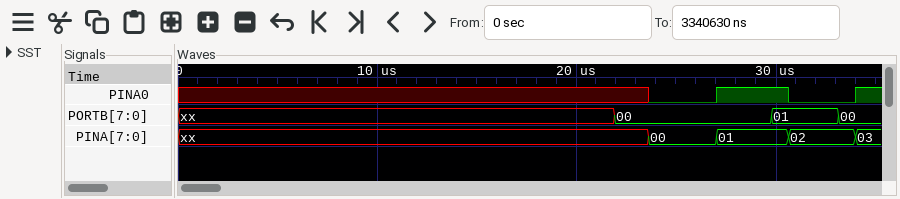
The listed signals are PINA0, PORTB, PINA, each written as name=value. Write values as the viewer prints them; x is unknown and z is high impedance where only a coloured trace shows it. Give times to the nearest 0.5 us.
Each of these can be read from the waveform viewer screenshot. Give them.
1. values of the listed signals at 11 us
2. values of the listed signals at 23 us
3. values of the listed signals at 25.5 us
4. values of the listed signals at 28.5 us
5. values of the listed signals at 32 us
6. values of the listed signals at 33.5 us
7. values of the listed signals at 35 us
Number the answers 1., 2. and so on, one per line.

1. PINA0=x, PORTB=xx, PINA=xx
2. PINA0=x, PORTB=00, PINA=xx
3. PINA0=0, PORTB=00, PINA=00
4. PINA0=1, PORTB=00, PINA=01
5. PINA0=0, PORTB=01, PINA=02
6. PINA0=0, PORTB=00, PINA=02
7. PINA0=1, PORTB=00, PINA=03
